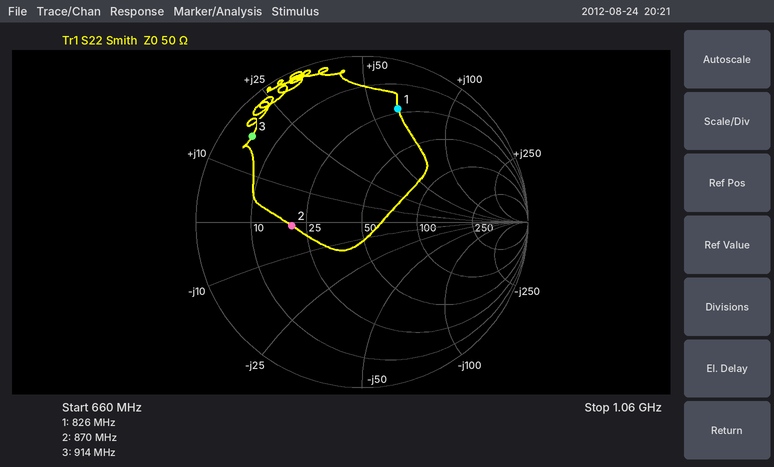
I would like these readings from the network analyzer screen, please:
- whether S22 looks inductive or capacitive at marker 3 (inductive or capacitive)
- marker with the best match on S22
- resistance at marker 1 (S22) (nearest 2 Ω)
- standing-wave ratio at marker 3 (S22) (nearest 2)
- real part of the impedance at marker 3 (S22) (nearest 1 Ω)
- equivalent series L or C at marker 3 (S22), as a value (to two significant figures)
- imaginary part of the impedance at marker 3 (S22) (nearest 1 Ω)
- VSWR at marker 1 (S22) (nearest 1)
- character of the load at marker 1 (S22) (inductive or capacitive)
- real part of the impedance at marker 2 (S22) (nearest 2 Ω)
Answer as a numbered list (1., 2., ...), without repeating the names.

1. inductive
2. marker 2
3. 22 Ω
4. 12
5. 5 Ω
6. 3.0 nH
7. +17 Ω
8. 6
9. inductive
10. 20 Ω
